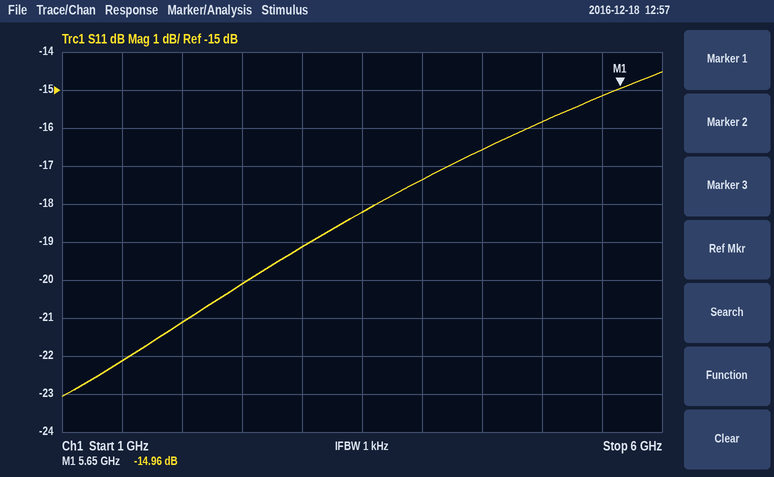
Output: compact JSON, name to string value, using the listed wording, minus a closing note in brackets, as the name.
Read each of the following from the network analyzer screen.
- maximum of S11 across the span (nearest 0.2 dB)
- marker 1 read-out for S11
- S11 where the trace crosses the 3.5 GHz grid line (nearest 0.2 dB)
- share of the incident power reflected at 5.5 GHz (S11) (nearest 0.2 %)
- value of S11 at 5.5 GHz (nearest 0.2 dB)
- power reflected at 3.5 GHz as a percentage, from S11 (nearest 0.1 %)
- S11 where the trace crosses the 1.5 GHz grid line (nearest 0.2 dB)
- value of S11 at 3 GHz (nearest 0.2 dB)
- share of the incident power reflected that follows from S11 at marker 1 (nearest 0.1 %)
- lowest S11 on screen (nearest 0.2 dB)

{"maximum of S11 across the span": "-14.6 dB", "marker 1 read-out for S11": "-14.96 dB", "S11 where the trace crosses the 3.5 GHz grid line": "-18.2 dB", "share of the incident power reflected at 5.5 GHz (S11)": "3.0 %", "value of S11 at 5.5 GHz": "-15.2 dB", "power reflected at 3.5 GHz as a percentage, from S11": "1.5 %", "S11 where the trace crosses the 1.5 GHz grid line": "-22.2 dB", "value of S11 at 3 GHz": "-19.2 dB", "share of the incident power reflected that follows from S11 at marker 1": "3.2 %", "lowest S11 on screen": "-23.0 dB"}
